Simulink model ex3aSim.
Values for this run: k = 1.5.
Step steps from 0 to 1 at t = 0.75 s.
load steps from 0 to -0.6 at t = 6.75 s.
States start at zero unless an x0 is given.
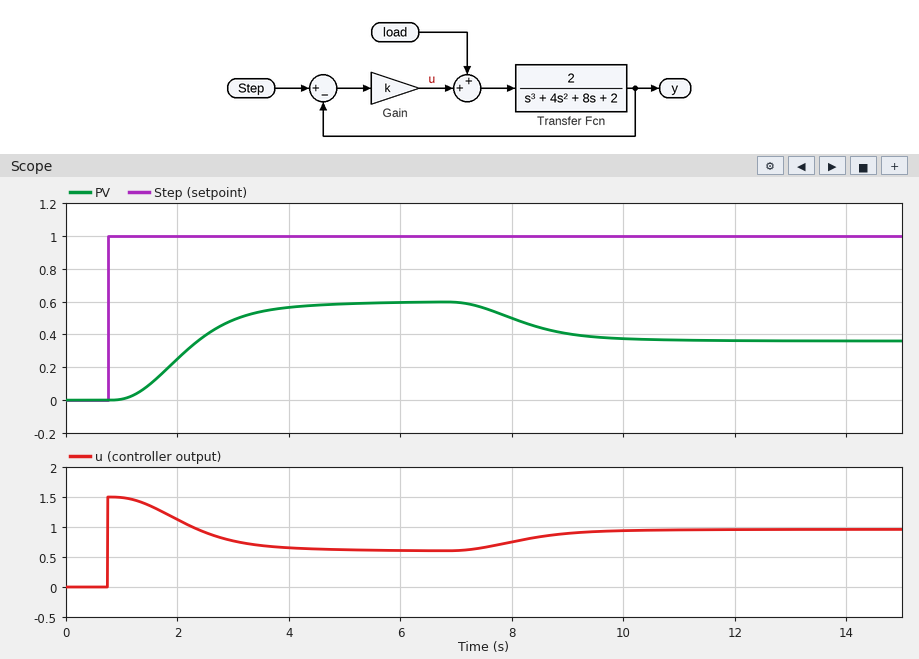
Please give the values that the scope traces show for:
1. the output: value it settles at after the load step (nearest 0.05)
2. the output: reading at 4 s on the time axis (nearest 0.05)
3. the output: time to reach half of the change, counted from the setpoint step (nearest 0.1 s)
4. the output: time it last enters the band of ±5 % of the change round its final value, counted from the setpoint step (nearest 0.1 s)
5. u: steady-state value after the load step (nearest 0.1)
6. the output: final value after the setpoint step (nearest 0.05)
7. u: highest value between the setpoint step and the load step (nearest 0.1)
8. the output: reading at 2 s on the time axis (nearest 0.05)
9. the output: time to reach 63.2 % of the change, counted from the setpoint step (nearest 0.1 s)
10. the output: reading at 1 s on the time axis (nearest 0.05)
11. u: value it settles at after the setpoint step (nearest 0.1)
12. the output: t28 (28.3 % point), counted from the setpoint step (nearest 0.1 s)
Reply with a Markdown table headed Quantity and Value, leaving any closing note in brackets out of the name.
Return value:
| Quantity | Value |
|---|---|
| the output: value it settles at after the load step | 0.35 |
| the output: reading at 4 s on the time axis | 0.55 |
| the output: time to reach half of the change, counted from the setpoint step | 1.4 s |
| the output: time it last enters the band of ±5 % of the change round its final value, counted from the setpoint step | 3.4 s |
| u: steady-state value after the load step | 1.0 |
| the output: final value after the setpoint step | 0.60 |
| u: highest value between the setpoint step and the load step | 1.5 |
| the output: reading at 2 s on the time axis | 0.25 |
| the output: time to reach 63.2 % of the change, counted from the setpoint step | 1.7 s |
| the output: reading at 1 s on the time axis | 0.00 |
| u: value it settles at after the setpoint step | 0.6 |
| the output: t28 (28.3 % point), counted from the setpoint step | 1.0 s |
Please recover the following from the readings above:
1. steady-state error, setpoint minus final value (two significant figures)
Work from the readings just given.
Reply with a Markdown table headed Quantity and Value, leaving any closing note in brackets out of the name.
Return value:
| Quantity | Value |
|---|---|
| steady-state error, setpoint minus final value | 0.40 |
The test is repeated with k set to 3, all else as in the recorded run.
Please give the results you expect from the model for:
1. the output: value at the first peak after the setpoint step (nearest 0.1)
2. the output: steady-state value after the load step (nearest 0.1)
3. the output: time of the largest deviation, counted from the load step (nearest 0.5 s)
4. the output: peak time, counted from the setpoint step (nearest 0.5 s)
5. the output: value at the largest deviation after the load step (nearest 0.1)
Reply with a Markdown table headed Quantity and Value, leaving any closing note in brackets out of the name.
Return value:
| Quantity | Value |
|---|---|
| the output: value at the first peak after the setpoint step | 0.8 |
| the output: steady-state value after the load step | 0.6 |
| the output: time of the largest deviation, counted from the load step | 2.5 s |
| the output: peak time, counted from the setpoint step | 2.5 s |
| the output: value at the largest deviation after the load step | 0.6 |
